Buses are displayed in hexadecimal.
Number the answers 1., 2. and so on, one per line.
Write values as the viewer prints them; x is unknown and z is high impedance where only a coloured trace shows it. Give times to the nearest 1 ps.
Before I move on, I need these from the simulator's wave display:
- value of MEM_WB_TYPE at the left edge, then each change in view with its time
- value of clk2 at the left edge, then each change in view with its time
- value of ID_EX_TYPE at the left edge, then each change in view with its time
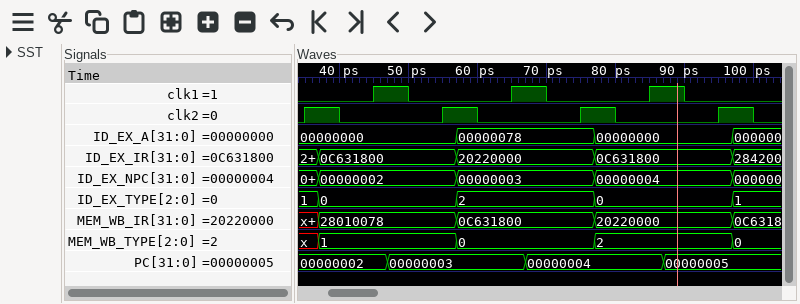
1. x, 1 at 37 ps, 0 at 57 ps, 2 at 77 ps, 0 at 97 ps
2. 0, 1 at 35 ps, 0 at 40 ps, 1 at 55 ps, 0 at 60 ps, 1 at 75 ps, 0 at 80 ps, 1 at 95 ps, 0 at 100 ps
3. 1, 0 at 37 ps, 2 at 57 ps, 0 at 77 ps, 1 at 97 ps
